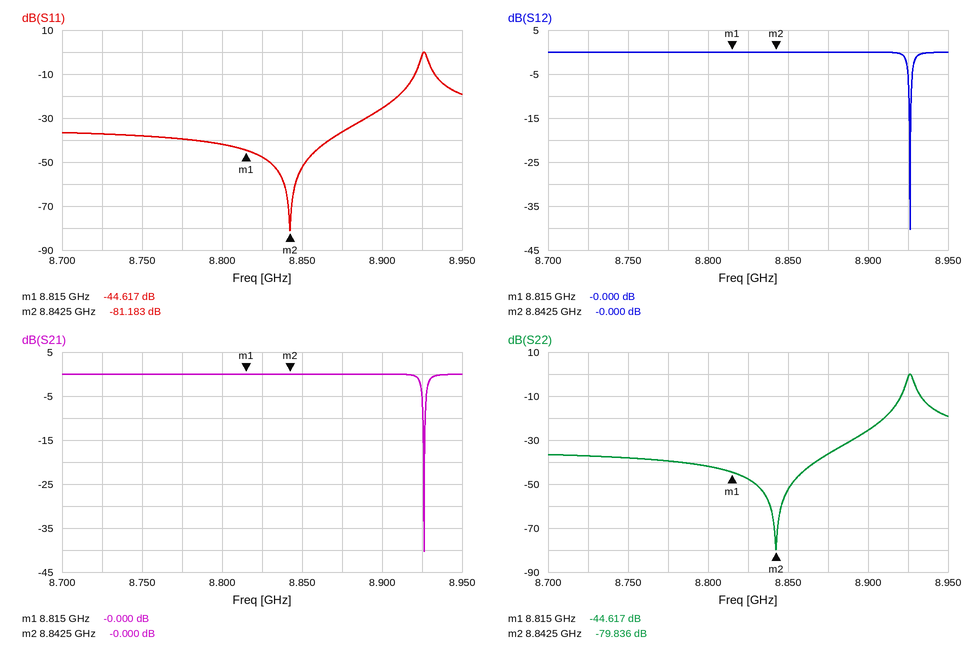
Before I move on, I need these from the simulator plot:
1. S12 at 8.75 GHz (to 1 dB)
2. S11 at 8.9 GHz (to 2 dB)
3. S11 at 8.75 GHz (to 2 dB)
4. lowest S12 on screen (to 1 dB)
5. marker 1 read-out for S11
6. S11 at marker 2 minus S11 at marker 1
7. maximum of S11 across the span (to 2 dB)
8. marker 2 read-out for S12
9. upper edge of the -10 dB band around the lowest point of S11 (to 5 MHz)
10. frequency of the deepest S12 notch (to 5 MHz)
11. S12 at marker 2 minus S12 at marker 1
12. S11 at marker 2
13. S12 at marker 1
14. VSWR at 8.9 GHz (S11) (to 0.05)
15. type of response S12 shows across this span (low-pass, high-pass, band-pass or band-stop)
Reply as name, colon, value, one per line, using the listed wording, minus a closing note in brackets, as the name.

S12 at 8.75 GHz: 0 dB
S11 at 8.9 GHz: -26 dB
S11 at 8.75 GHz: -38 dB
lowest S12 on screen: -40 dB
marker 1 read-out for S11: -44.617 dB
S11 at marker 2 minus S11 at marker 1: -36.566 dB
maximum of S11 across the span: 0 dB
marker 2 read-out for S12: -0.000 dB
upper edge of the -10 dB band around the lowest point of S11: 8.920 GHz
frequency of the deepest S12 notch: 8.925 GHz
S12 at marker 2 minus S12 at marker 1: 0.000 dB
S11 at marker 2: -81.183 dB
S12 at marker 1: -0.000 dB
VSWR at 8.9 GHz (S11): 1.10
type of response S12 shows across this span: band-stop
